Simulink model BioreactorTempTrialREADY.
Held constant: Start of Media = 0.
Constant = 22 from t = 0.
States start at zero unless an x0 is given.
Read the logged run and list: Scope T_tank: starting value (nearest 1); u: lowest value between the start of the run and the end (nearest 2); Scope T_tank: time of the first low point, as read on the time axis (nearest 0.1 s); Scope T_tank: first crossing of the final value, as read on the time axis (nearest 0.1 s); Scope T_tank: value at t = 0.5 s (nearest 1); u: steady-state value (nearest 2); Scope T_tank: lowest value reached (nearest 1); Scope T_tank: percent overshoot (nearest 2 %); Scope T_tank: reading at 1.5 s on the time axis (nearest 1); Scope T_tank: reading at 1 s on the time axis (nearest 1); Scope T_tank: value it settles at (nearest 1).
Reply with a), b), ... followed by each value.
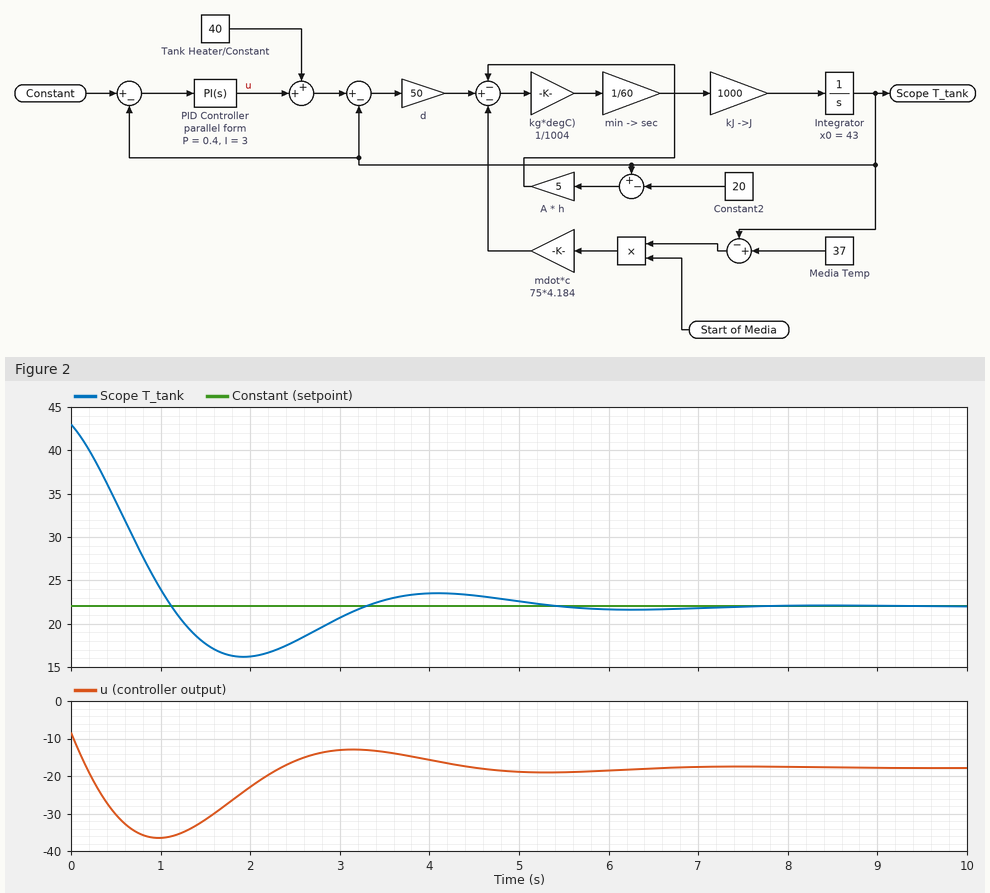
a) 43
b) -36
c) 1.9 s
d) 1.1 s
e) 34
f) -18
g) 16
h) 28 %
i) 18
j) 24
k) 22
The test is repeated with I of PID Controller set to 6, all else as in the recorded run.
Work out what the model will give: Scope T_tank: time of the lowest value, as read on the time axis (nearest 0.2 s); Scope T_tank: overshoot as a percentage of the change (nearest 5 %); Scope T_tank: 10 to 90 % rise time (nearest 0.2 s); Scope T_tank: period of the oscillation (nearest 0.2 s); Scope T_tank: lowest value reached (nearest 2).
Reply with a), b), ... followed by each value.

a) 1.4 s
b) 40 %
c) 0.6 s
d) 3.0 s
e) 14
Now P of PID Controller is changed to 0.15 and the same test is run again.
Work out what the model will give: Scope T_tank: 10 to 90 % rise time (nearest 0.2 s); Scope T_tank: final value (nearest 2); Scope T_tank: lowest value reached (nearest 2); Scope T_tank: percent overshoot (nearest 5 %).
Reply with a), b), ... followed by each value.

a) 0.8 s
b) 22
c) 14
d) 35 %
